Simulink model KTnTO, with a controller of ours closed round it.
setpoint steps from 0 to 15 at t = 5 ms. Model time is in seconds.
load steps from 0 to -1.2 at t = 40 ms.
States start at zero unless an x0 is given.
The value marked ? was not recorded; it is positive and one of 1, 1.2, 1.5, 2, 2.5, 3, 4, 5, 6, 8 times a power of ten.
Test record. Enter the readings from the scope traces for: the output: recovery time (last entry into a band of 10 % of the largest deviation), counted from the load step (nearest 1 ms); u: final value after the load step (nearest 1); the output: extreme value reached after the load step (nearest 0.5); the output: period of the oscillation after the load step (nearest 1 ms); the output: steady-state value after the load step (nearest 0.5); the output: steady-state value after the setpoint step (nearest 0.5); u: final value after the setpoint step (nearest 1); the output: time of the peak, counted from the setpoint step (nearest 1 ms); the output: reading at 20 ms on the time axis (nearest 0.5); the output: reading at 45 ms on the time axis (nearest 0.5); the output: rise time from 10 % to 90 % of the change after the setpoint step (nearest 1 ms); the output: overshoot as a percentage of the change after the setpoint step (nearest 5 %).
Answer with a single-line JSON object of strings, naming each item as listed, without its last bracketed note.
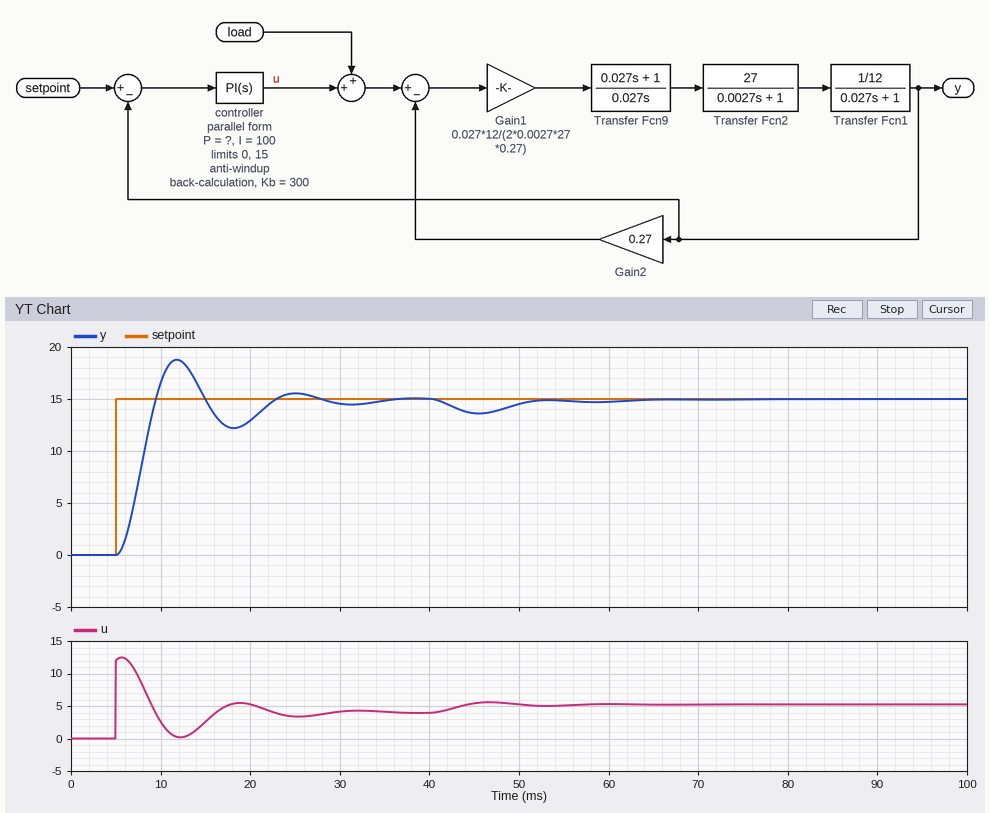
{"the output: recovery time (last entry into a band of 10 % of the largest deviation), counted from the load step": "23 ms", "u: final value after the load step": "5", "the output: extreme value reached after the load step": "13.5", "the output: period of the oscillation after the load step": "13 ms", "the output: steady-state value after the load step": "15.0", "the output: steady-state value after the setpoint step": "15.0", "u: final value after the setpoint step": "4", "the output: time of the peak, counted from the setpoint step": "7 ms", "the output: reading at 20 ms on the time axis": "13.0", "the output: reading at 45 ms on the time axis": "13.5", "the output: rise time from 10 % to 90 % of the change after the setpoint step": "3 ms", "the output: overshoot as a percentage of the change after the setpoint step": "25 %"}
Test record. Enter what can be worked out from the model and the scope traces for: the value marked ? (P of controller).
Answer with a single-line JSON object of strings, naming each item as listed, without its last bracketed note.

{"the value marked ?": "0.8"}
